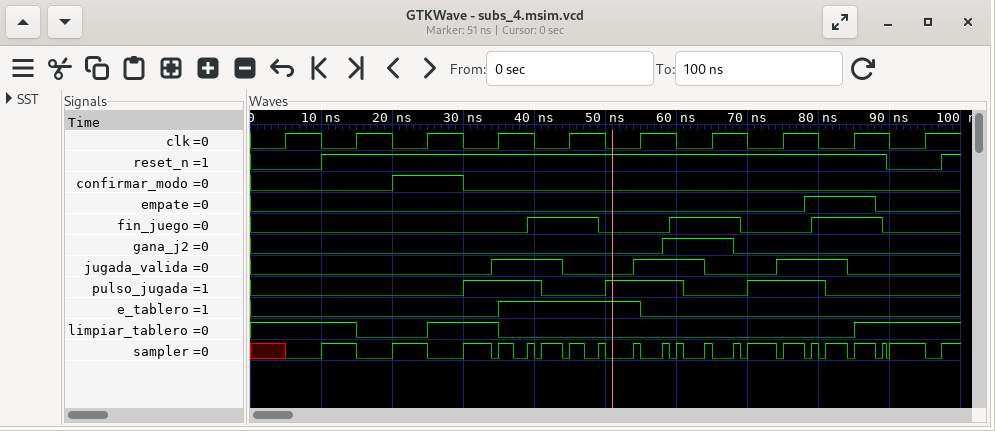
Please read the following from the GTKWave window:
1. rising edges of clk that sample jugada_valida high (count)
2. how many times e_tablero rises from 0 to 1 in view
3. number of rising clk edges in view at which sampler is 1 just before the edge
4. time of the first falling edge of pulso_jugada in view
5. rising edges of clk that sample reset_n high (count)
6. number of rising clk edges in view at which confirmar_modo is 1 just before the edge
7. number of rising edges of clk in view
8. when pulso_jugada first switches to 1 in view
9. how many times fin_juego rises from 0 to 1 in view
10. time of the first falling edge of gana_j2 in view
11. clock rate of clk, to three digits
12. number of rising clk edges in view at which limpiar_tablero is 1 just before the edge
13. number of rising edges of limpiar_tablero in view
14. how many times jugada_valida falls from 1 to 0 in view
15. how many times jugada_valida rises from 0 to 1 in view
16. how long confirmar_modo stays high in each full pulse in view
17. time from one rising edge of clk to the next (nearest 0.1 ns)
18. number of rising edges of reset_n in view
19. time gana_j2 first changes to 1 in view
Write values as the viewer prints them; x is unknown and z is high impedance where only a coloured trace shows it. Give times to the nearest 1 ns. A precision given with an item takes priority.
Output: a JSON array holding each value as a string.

["3", "1", "5", "41 ns", "8", "1", "10", "30 ns", "3", "68 ns", "100 MHz", "4", "2", "3", "3", "10 ns", "10 ns", "2", "58 ns"]
